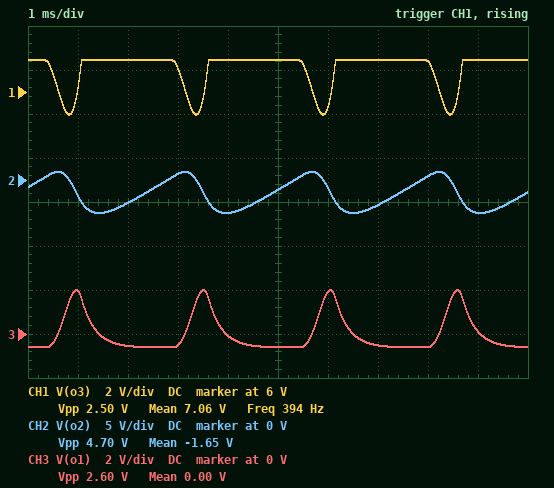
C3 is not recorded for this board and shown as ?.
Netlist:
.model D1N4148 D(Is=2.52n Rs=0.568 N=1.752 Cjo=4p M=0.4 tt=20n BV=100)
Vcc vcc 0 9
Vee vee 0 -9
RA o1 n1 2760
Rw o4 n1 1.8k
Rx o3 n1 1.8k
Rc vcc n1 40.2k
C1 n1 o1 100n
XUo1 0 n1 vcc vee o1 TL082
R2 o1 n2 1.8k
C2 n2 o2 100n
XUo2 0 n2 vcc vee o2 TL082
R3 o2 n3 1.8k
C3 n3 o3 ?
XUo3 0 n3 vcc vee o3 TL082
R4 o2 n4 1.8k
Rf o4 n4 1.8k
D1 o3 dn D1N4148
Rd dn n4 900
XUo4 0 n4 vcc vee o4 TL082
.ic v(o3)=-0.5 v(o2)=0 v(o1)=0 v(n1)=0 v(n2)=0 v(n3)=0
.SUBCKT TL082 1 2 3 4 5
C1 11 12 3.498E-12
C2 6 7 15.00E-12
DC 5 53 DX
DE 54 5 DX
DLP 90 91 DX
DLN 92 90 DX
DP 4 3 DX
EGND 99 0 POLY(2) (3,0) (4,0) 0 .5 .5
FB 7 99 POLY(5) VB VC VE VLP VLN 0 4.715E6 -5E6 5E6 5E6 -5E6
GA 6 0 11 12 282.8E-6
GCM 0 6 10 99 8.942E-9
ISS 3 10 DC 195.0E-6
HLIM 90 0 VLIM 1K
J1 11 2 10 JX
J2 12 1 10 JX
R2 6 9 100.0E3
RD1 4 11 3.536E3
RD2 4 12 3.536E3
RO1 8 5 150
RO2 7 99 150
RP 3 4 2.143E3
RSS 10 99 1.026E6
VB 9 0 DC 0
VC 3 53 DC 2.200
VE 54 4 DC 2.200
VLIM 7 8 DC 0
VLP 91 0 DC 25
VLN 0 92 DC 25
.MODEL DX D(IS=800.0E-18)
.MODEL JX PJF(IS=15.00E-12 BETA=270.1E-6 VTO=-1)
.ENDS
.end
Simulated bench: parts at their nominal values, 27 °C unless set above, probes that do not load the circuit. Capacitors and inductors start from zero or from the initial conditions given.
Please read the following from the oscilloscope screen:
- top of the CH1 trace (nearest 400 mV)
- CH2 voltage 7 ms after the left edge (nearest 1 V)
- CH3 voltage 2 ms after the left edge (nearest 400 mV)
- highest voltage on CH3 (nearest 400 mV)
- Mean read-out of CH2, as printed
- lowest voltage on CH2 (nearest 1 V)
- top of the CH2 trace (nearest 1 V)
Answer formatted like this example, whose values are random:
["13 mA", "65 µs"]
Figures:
["7.6 V", "-3 V", "-400 mV", "2.0 V", "-1.65 V", "-4 V", "1 V"]
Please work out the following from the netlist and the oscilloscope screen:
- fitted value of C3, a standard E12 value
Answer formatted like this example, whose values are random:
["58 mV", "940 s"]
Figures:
["68 nF"]
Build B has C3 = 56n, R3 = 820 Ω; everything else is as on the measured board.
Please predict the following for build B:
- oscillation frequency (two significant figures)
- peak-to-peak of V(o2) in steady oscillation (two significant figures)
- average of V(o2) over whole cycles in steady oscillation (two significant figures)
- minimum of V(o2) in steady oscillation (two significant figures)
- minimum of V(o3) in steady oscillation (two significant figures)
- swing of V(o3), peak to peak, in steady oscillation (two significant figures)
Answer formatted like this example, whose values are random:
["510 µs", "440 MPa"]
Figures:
["480 Hz", "3.7 V", "-1.5 V", "-3.1 V", "4.5 V", "3.0 V"]
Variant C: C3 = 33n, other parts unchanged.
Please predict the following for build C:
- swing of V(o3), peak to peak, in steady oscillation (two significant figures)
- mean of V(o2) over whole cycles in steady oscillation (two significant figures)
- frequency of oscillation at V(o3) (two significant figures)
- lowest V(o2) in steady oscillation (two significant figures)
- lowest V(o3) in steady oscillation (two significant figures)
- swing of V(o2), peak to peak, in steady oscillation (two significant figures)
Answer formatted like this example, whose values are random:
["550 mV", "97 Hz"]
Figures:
["2.8 V", "-1.5 V", "460 Hz", "-3.2 V", "4.7 V", "3.9 V"]
